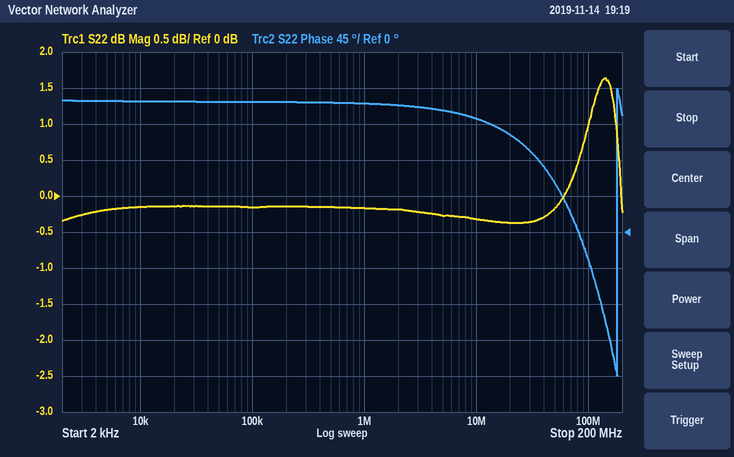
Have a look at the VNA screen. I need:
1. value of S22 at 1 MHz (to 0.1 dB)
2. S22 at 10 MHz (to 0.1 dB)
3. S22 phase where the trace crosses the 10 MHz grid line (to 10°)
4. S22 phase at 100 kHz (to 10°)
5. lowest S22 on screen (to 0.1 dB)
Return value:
-0.2 dB
-0.3 dB
140°
160°
-0.4 dB
